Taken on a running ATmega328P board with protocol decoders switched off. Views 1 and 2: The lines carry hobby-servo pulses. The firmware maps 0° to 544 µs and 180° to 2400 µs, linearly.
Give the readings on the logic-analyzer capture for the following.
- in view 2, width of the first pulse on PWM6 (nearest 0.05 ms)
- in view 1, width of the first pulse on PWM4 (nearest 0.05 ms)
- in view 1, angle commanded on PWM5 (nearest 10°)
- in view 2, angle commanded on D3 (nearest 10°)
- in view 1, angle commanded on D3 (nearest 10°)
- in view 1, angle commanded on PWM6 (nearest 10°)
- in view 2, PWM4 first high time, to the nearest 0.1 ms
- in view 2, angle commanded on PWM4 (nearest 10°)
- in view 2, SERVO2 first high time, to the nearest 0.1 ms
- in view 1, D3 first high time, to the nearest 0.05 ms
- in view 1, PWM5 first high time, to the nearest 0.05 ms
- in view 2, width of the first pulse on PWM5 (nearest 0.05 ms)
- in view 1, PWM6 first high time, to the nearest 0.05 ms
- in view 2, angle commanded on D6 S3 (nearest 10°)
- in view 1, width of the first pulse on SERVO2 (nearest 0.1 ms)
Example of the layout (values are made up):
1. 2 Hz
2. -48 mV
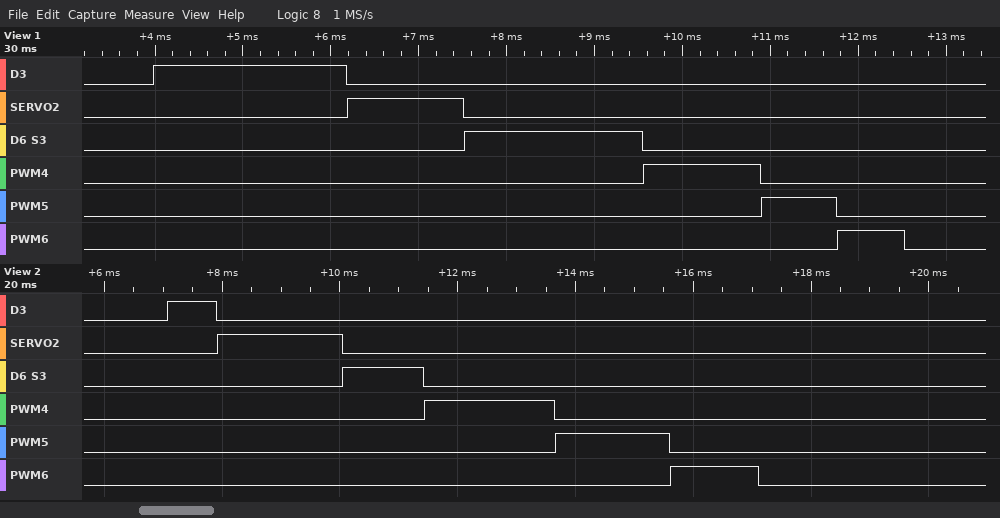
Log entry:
1. 1.50 ms
2. 1.35 ms
3. 30°
4. 30°
5. 160°
6. 20°
7. 2.2 ms
8. 160°
9. 2.1 ms
10. 2.20 ms
11. 0.85 ms
12. 1.95 ms
13. 0.75 ms
14. 80°
15. 1.3 ms
